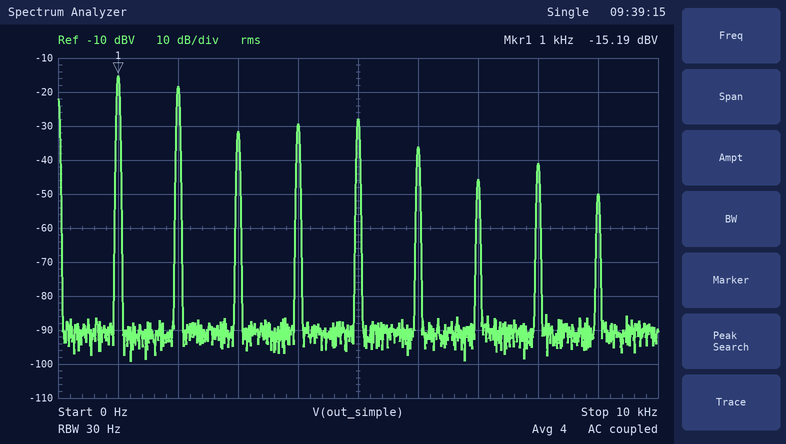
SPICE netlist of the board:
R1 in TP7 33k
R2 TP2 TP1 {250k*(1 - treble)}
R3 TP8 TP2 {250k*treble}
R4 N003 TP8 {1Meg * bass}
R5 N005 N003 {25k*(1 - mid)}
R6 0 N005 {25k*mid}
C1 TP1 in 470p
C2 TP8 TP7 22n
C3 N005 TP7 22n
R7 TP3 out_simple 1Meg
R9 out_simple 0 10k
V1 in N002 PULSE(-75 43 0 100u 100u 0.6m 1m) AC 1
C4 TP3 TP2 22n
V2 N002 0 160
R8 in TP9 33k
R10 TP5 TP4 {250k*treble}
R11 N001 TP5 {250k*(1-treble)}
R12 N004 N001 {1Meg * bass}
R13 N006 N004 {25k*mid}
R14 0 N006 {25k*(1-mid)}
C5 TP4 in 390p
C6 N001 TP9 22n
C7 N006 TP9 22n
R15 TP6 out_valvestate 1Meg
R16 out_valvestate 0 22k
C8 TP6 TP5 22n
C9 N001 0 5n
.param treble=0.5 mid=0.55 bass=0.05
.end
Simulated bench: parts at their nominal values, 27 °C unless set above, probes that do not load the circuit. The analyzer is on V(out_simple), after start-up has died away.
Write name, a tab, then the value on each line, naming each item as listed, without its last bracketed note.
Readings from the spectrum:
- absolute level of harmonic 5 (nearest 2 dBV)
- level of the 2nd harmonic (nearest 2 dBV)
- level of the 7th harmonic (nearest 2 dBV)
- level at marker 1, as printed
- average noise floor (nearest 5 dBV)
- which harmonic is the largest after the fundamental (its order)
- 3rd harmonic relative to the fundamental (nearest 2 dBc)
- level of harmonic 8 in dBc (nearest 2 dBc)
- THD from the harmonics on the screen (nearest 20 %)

absolute level of harmonic 5	-28 dBV
level of the 2nd harmonic	-18 dBV
level of the 7th harmonic	-46 dBV
level at marker 1, as printed	-15.19 dBV
average noise floor	-90 dBV
which harmonic is the largest after the fundamental	2
3rd harmonic relative to the fundamental	-16 dBc
level of harmonic 8 in dBc	-26 dBc
THD from the harmonics on the screen	80 %
